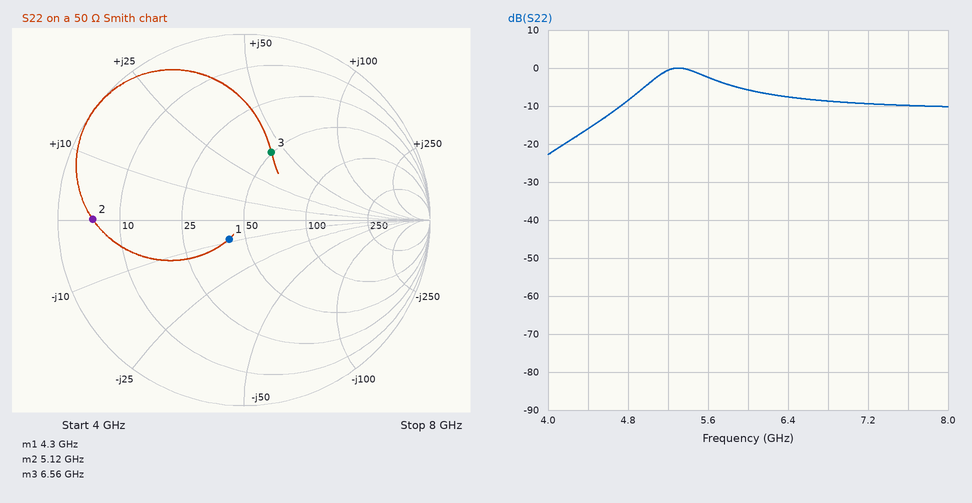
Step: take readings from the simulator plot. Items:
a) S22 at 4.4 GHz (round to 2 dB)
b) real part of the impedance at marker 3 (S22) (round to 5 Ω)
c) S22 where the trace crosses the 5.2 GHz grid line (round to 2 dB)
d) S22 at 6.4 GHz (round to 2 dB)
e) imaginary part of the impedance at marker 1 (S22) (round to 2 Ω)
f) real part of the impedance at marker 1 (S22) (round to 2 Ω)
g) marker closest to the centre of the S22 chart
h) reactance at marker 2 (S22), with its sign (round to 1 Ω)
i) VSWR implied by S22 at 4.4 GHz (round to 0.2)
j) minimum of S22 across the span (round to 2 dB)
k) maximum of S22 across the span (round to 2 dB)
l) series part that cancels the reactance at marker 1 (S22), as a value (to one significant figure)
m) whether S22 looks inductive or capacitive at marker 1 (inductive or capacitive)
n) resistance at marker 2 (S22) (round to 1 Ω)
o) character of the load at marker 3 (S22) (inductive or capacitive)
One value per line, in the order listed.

-16 dB
50 Ω
0 dB
-8 dB
-8 Ω
42 Ω
marker 1
0 Ω
1.4
-22 dB
0 dB
300 pH
capacitive
5 Ω
inductive
